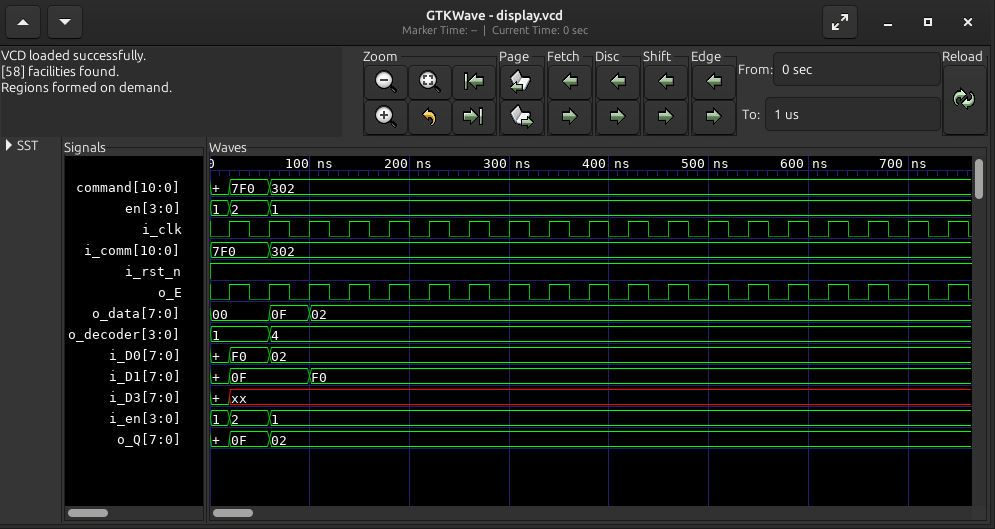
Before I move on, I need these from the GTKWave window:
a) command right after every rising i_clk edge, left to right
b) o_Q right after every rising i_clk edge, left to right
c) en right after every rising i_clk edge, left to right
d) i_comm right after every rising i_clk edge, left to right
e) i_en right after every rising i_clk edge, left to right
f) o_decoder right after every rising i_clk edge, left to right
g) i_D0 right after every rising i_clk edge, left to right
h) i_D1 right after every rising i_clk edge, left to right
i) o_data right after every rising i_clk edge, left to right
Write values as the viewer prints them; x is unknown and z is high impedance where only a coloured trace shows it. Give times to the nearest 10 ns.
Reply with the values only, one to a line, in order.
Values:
7F0, 302, 302, 302, 302, 302, 302, 302, 302, 302, 302, 302, 302, 302, 302, 302, 302, 302, 302
0F, 02, 02, 02, 02, 02, 02, 02, 02, 02, 02, 02, 02, 02, 02, 02, 02, 02, 02
2, 1, 1, 1, 1, 1, 1, 1, 1, 1, 1, 1, 1, 1, 1, 1, 1, 1, 1
7F0, 302, 302, 302, 302, 302, 302, 302, 302, 302, 302, 302, 302, 302, 302, 302, 302, 302, 302
2, 1, 1, 1, 1, 1, 1, 1, 1, 1, 1, 1, 1, 1, 1, 1, 1, 1, 1
1, 4, 4, 4, 4, 4, 4, 4, 4, 4, 4, 4, 4, 4, 4, 4, 4, 4, 4
F0, 02, 02, 02, 02, 02, 02, 02, 02, 02, 02, 02, 02, 02, 02, 02, 02, 02, 02
0F, 0F, F0, F0, F0, F0, F0, F0, F0, F0, F0, F0, F0, F0, F0, F0, F0, F0, F0
00, 0F, 02, 02, 02, 02, 02, 02, 02, 02, 02, 02, 02, 02, 02, 02, 02, 02, 02
